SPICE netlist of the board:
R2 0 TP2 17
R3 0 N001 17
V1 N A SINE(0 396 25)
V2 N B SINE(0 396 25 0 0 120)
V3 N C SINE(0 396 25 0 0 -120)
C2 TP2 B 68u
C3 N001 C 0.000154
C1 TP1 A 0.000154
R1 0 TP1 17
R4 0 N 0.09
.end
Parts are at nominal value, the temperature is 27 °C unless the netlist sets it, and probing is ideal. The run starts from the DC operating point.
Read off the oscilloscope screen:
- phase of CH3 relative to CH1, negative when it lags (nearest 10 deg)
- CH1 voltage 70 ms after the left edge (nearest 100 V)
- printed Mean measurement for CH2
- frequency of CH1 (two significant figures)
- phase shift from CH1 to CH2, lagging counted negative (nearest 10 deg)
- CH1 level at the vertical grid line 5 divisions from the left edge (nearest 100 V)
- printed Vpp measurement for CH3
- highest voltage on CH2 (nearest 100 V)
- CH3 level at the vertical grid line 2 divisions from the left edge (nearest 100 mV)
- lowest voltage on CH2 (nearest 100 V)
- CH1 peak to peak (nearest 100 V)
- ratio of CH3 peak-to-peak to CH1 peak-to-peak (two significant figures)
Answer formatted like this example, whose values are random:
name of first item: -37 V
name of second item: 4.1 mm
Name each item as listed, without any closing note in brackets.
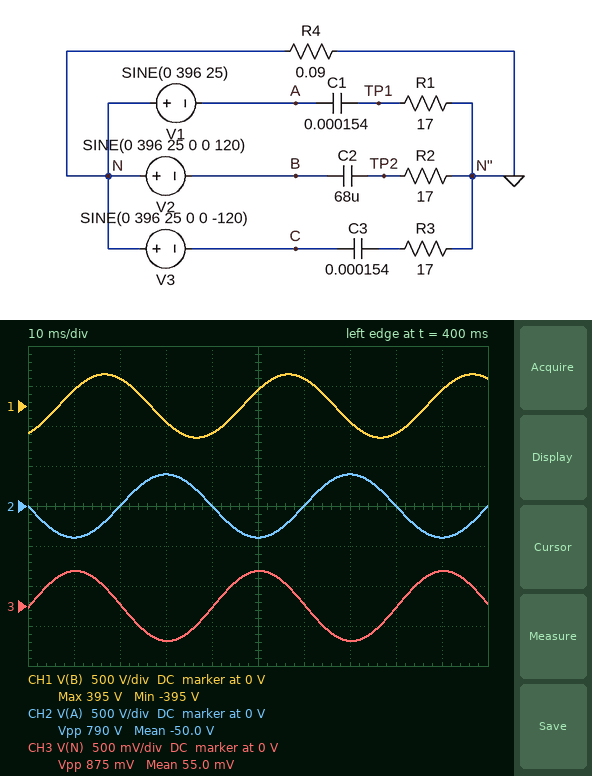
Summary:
phase of CH3 relative to CH1, negative when it lags: 60 deg
CH1 voltage 70 ms after the left edge: -200 V
printed Mean measurement for CH2: -50.0 V
frequency of CH1: 25 Hz
phase shift from CH1 to CH2, lagging counted negative: -120 deg
CH1 level at the vertical grid line 5 divisions from the left edge: 200 V
printed Vpp measurement for CH3: 875 mV
highest voltage on CH2: 400 V
CH3 level at the vertical grid line 2 divisions from the left edge: 0 V
lowest voltage on CH2: -400 V
CH1 peak to peak: 800 V
ratio of CH3 peak-to-peak to CH1 peak-to-peak: 0.0011
